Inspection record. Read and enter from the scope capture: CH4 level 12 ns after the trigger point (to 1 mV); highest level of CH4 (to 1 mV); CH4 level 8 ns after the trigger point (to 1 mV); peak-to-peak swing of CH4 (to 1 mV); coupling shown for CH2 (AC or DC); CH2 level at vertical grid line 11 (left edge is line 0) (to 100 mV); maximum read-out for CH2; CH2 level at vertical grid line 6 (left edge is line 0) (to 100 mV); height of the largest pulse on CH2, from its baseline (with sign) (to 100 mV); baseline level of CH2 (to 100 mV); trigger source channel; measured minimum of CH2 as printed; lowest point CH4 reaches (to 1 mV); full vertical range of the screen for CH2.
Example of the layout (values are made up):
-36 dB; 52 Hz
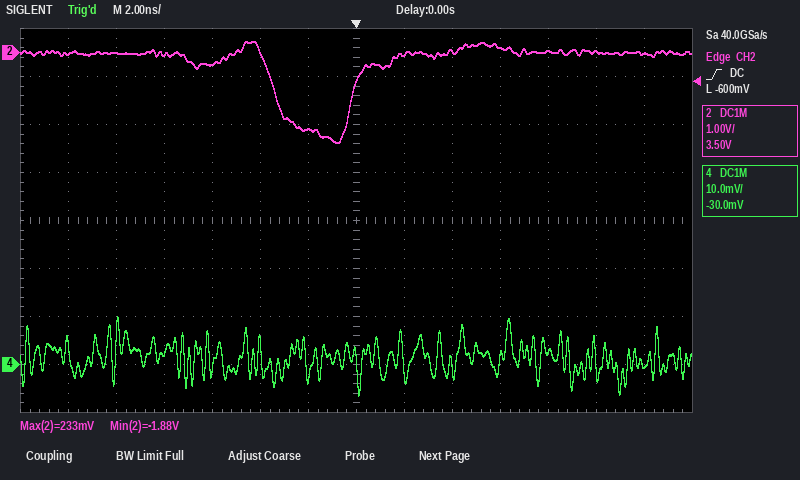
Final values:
0 mV; 10 mV; 3 mV; 16 mV; DC; 0.0 V; 233 mV; -1.6 V; -1.9 V; 0.0 V; CH2; -1.88 V; -6 mV; 8 V
